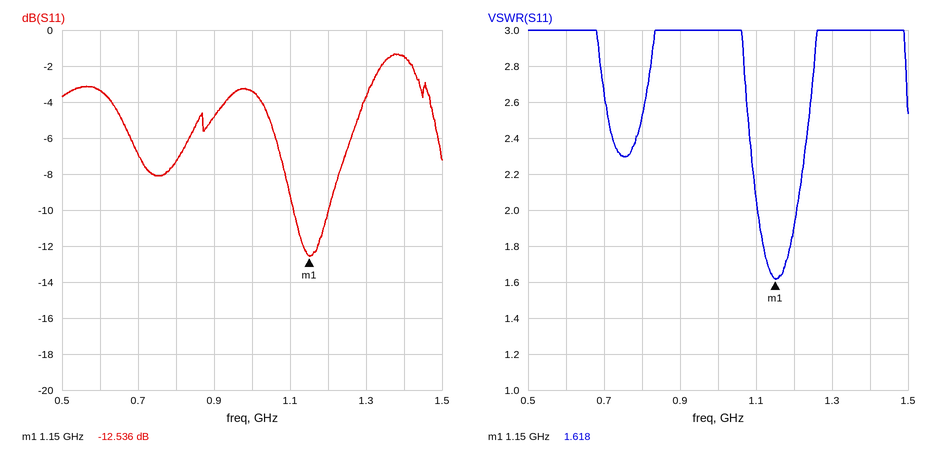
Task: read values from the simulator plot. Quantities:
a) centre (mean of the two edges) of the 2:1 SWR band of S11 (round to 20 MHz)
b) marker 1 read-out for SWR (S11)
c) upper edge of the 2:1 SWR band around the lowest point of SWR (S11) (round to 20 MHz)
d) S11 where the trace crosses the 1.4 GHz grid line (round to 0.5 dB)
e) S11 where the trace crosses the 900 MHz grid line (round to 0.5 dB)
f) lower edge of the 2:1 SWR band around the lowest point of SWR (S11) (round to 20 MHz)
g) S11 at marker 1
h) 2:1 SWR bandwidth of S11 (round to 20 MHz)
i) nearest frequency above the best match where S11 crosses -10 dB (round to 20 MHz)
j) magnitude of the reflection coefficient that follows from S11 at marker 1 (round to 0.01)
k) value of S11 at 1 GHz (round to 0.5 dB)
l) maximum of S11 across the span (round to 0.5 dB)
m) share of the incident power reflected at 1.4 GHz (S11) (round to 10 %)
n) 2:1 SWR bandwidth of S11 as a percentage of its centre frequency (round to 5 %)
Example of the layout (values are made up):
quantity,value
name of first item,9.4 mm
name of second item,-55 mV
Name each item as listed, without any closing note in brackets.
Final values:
quantity,value
centre (mean of the two edges) of the 2:1 SWR band of S11,1.16 GHz
marker 1 read-out for SWR,1.618
upper edge of the 2:1 SWR band around the lowest point of SWR (S11),1.20 GHz
S11 where the trace crosses the 1.4 GHz grid line,-1.5 dB
S11 where the trace crosses the 900 MHz grid line,-5.0 dB
lower edge of the 2:1 SWR band around the lowest point of SWR (S11),1.10 GHz
S11 at marker 1,-12.536 dB
2:1 SWR bandwidth of S11,100 MHz
nearest frequency above the best match where S11 crosses -10 dB,1.20 GHz
magnitude of the reflection coefficient that follows from S11 at marker 1,0.24
value of S11 at 1 GHz,-3.5 dB
maximum of S11 across the span,-1.5 dB
share of the incident power reflected at 1.4 GHz (S11),70 %
2:1 SWR bandwidth of S11 as a percentage of its centre frequency,10 %
